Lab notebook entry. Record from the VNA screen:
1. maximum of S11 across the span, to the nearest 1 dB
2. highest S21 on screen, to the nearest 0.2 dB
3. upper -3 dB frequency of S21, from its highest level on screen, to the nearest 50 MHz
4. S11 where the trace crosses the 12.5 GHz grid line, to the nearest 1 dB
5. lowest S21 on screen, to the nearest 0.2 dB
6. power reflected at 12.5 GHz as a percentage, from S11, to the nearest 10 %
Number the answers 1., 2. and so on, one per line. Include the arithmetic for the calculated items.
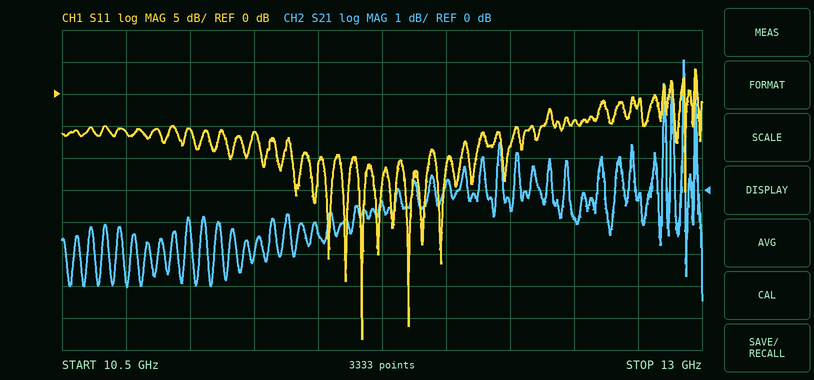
1. 4 dB
2. 4.0 dB
3. 12.95 GHz
4. -4 dB
5. -3.4 dB
6. 10^(-4/10) ≈ 40 %
